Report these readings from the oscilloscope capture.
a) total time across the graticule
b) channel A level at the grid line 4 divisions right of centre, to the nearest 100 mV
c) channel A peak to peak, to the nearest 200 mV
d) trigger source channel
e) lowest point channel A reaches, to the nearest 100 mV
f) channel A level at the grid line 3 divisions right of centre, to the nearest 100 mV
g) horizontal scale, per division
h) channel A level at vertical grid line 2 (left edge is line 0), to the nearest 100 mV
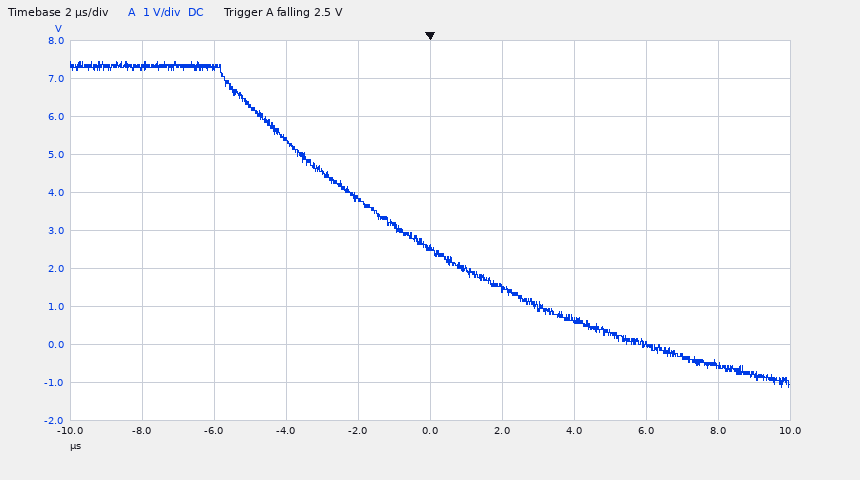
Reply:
20 µs
-600 mV
8.6 V
channel A
-1.1 V
0.0 V
2 µs
7.3 V
